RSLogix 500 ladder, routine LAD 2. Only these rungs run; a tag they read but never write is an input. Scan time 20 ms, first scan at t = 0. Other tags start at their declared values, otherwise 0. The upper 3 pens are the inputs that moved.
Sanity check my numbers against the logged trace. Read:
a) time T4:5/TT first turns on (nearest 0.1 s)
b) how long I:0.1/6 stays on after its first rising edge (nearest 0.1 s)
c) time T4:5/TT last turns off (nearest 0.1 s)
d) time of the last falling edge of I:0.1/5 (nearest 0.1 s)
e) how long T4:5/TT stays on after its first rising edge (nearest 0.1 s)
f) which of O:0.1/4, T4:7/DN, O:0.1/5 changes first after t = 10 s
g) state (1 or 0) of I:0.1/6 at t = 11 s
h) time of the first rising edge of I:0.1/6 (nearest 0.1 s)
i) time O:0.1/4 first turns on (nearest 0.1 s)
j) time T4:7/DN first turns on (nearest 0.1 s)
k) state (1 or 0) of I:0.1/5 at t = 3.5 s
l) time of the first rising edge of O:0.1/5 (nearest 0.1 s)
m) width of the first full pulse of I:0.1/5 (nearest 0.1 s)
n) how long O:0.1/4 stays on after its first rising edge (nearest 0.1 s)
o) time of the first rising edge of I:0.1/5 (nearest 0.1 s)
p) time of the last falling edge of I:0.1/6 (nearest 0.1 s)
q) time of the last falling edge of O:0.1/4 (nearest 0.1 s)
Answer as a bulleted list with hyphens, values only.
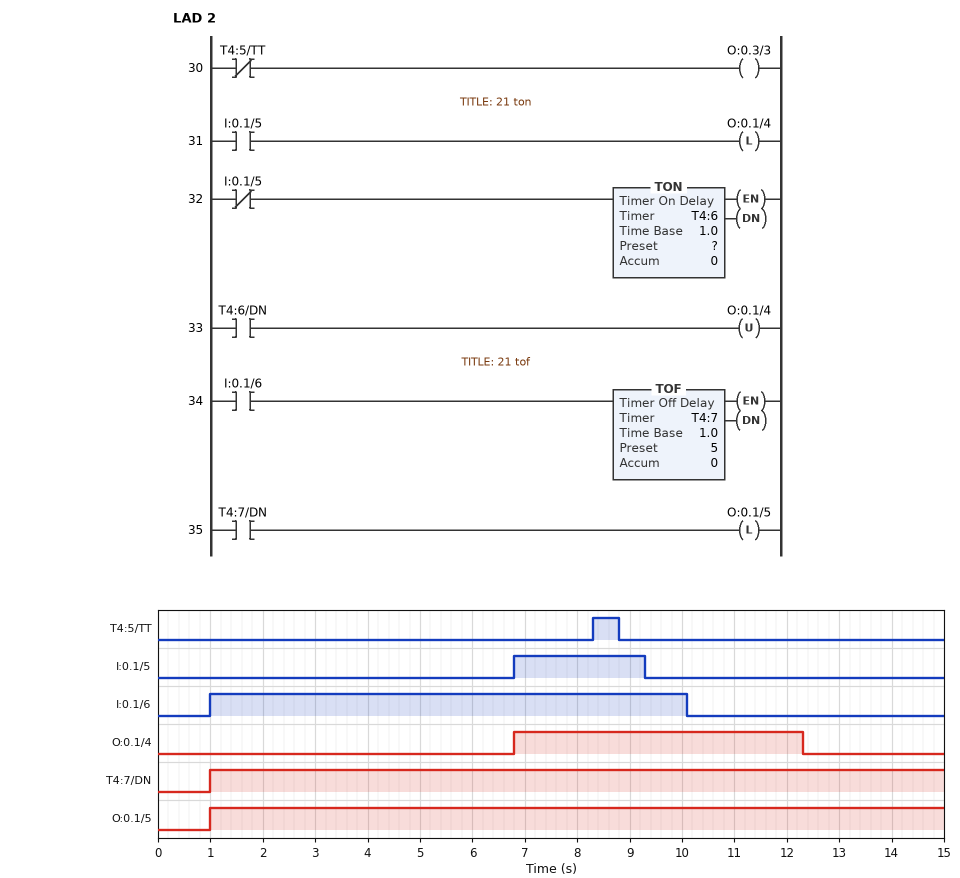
- 8.3 s
- 9.1 s
- 8.8 s
- 9.3 s
- 0.5 s
- O:0.1/4
- 0
- 1.0 s
- 6.8 s
- 1.0 s
- 0
- 1.0 s
- 2.5 s
- 5.5 s
- 6.8 s
- 10.1 s
- 12.3 s
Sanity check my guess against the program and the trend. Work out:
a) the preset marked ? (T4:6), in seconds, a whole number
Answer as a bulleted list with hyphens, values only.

- 3 s
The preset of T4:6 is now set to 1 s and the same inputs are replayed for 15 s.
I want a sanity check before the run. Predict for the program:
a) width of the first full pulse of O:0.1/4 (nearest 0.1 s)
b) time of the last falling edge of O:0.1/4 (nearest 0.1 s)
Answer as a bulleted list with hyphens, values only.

- 3.5 s
- 10.3 s
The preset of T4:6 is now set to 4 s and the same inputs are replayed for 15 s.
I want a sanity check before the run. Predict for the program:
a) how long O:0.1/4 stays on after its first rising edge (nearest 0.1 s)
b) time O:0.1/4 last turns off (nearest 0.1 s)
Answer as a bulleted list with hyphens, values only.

- 6.5 s
- 13.3 s
